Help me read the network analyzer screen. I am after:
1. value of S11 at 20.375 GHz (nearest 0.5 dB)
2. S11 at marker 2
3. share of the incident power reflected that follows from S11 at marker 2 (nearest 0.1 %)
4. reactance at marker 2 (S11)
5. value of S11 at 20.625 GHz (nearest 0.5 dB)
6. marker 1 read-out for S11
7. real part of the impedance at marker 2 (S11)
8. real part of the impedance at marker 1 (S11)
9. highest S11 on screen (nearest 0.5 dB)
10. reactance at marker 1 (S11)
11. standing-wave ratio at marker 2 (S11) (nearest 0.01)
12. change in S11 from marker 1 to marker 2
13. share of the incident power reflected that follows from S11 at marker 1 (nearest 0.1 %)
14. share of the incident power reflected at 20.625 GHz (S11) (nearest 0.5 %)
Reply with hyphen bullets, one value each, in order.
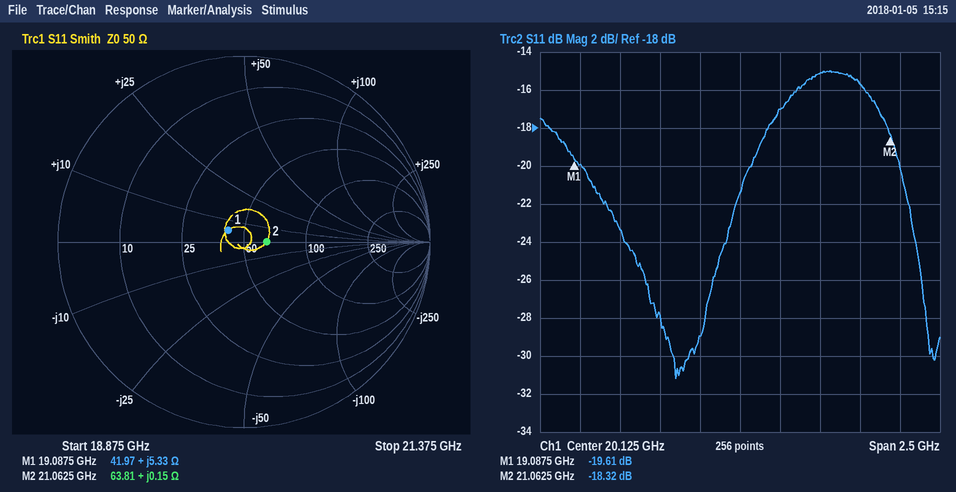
- -17.0 dB
- -18.32 dB
- 1.5 %
- +0.15 Ω
- -15.0 dB
- -19.61 dB
- 63.81 Ω
- 41.97 Ω
- -15.0 dB
- +5.33 Ω
- 1.28
- 1.29 dB
- 1.1 %
- 3.0 %
